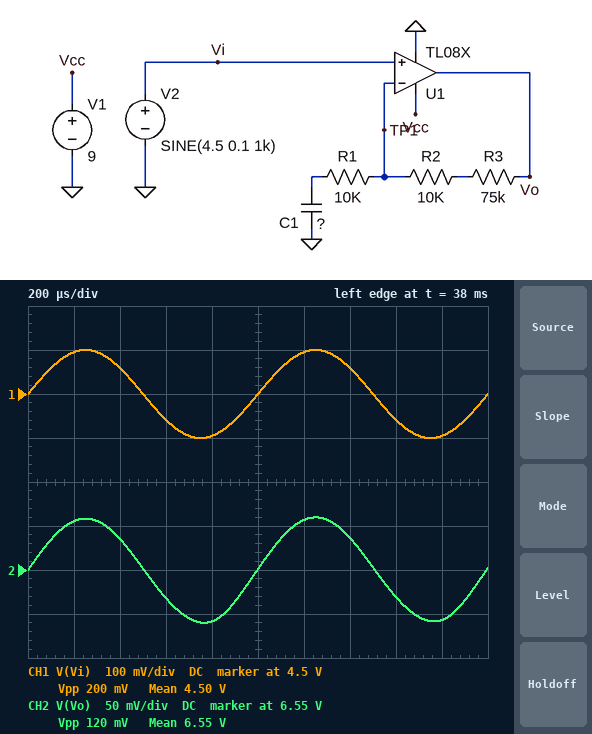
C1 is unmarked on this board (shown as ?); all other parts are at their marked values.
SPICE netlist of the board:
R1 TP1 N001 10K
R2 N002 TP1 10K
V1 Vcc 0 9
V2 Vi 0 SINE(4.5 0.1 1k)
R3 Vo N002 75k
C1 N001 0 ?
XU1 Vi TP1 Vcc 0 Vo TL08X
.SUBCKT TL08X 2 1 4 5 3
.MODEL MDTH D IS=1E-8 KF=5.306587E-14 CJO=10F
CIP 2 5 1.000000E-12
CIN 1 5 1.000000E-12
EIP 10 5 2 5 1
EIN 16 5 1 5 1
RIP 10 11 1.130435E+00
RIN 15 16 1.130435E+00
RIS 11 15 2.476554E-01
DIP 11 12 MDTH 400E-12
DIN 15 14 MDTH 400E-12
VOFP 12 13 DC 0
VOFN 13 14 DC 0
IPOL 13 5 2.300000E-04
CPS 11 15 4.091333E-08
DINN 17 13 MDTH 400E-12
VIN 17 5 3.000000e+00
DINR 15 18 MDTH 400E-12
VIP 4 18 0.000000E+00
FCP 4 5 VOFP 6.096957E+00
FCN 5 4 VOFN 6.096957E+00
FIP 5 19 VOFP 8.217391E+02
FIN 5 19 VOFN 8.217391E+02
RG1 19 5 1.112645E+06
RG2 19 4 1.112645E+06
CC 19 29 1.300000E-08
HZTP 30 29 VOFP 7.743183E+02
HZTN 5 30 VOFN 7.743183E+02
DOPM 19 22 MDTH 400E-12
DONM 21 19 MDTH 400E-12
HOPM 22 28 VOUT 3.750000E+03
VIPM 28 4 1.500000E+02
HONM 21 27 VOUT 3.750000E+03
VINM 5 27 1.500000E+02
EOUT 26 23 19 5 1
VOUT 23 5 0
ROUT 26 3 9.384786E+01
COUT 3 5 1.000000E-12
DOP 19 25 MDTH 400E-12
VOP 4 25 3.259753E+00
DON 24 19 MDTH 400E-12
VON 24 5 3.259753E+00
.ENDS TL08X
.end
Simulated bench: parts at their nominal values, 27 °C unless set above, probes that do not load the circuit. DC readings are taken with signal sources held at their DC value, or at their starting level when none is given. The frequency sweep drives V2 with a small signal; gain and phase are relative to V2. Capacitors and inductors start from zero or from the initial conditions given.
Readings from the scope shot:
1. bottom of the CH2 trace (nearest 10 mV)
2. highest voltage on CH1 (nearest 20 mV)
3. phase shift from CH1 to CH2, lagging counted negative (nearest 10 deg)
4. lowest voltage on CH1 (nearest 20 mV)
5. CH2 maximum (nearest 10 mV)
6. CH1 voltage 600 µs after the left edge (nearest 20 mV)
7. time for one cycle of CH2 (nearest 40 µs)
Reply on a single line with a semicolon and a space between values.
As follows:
6.49 V; 4.60 V; 0 deg; 4.40 V; 6.61 V; 4.44 V; 1.00 ms
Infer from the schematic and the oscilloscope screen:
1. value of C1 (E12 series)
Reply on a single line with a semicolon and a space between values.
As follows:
22 µF
